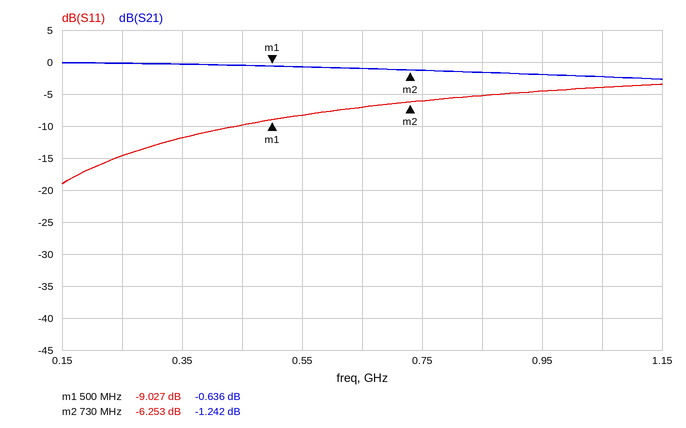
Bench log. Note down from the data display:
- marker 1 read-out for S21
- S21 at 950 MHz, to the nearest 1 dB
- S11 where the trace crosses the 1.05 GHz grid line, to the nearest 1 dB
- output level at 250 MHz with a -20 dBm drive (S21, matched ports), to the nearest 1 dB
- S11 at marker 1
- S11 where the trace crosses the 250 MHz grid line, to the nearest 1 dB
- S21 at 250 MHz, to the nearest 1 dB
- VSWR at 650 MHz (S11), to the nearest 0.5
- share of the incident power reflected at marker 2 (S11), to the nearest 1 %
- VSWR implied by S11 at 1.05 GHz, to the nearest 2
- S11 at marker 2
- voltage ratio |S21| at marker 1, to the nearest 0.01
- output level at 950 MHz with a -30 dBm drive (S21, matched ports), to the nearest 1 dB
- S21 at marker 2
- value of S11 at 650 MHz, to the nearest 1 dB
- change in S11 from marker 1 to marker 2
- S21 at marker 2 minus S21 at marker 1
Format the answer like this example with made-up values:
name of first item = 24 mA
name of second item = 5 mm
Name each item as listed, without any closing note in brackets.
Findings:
marker 1 read-out for S21 = -0.636 dB
S21 at 950 MHz, to the nearest 1 dB = -2 dB
S11 where the trace crosses the 1.05 GHz grid line, to the nearest 1 dB = -4 dB
output level at 250 MHz with a -20 dBm drive (S21, matched ports), to the nearest 1 dB = -20 dBm
S11 at marker 1 = -9.027 dB
S11 where the trace crosses the 250 MHz grid line, to the nearest 1 dB = -15 dB
S21 at 250 MHz, to the nearest 1 dB = 0 dB
VSWR at 650 MHz (S11), to the nearest 0.5 = 2.5
share of the incident power reflected at marker 2 (S11), to the nearest 1 % = 24 %
VSWR implied by S11 at 1.05 GHz, to the nearest 2 = 4
S11 at marker 2 = -6.253 dB
voltage ratio |S21| at marker 1, to the nearest 0.01 = 0.93
output level at 950 MHz with a -30 dBm drive (S21, matched ports), to the nearest 1 dB = -32 dBm
S21 at marker 2 = -1.242 dB
value of S11 at 650 MHz, to the nearest 1 dB = -7 dB
change in S11 from marker 1 to marker 2 = 2.774 dB
S21 at marker 2 minus S21 at marker 1 = -0.606 dB
